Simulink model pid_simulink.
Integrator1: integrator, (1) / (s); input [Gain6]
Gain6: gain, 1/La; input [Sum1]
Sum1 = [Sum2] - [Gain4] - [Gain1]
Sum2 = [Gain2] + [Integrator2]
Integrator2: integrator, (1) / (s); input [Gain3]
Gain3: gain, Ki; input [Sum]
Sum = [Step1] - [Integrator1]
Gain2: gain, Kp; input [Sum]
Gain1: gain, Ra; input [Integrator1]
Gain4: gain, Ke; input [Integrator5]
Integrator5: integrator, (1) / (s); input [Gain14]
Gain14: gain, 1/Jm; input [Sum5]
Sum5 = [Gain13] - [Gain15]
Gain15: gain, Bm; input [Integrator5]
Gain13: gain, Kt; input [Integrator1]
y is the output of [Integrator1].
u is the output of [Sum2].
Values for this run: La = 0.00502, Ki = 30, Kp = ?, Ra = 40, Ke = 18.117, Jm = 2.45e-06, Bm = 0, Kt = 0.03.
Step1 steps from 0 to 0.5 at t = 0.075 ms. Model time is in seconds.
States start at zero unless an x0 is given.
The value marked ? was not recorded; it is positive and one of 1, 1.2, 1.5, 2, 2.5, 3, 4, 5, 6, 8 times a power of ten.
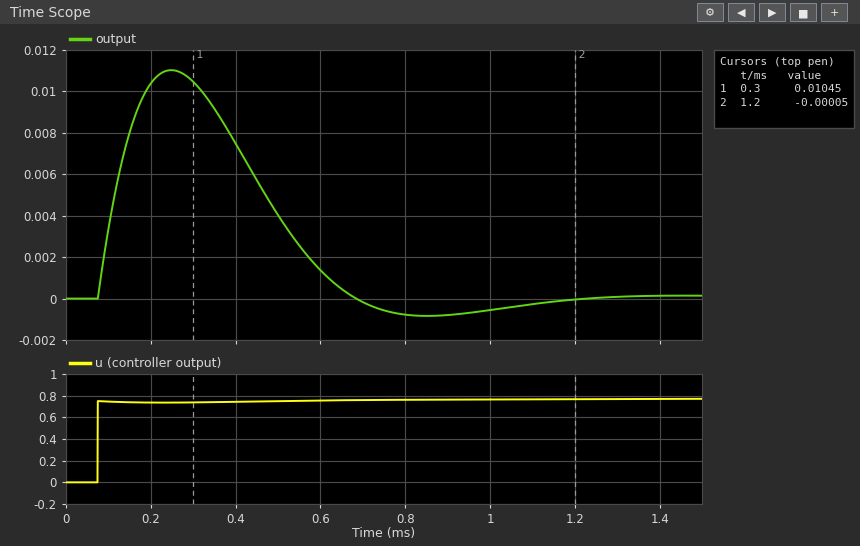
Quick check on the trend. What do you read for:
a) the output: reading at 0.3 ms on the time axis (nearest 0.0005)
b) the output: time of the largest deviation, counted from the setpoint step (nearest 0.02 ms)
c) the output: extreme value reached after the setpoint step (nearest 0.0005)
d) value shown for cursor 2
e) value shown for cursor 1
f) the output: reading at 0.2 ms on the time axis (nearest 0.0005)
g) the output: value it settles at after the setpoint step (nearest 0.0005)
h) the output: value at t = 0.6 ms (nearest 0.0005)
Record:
0.0105
0.18 ms
0.0110
-0.00005
0.01045
0.0105
0.0000
0.0015
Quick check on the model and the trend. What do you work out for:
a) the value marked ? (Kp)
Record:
1.5
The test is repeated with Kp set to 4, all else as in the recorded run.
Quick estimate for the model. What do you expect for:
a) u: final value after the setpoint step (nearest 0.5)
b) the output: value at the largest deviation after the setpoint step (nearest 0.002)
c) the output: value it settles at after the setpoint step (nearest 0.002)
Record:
2.0
0.028
0.000
